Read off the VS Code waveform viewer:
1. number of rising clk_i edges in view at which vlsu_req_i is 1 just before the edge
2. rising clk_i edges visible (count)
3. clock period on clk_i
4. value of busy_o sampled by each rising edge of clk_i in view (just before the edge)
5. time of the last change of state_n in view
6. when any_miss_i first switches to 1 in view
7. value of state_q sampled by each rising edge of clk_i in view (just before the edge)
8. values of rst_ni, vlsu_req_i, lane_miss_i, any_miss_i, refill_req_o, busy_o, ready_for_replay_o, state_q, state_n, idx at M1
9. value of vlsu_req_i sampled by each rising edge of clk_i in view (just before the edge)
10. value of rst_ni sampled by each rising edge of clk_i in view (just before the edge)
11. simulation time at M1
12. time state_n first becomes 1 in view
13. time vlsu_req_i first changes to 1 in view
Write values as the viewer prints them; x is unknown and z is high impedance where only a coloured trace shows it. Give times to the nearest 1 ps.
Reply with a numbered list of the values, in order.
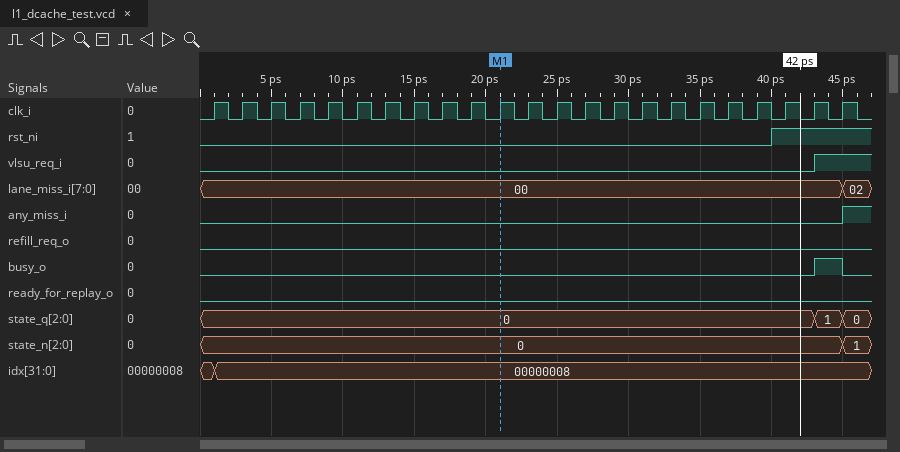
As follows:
1. 1
2. 23
3. 2 ps
4. 0 0 0 0 0 0 0 0 0 0 0 0 0 0 0 0 0 0 0 0 0 0 1
5. 45 ps
6. 45 ps
7. 0, 0, 0, 0, 0, 0, 0, 0, 0, 0, 0, 0, 0, 0, 0, 0, 0, 0, 0, 0, 0, 0, 1
8. rst_ni=0, vlsu_req_i=0, lane_miss_i=00, any_miss_i=0, refill_req_o=0, busy_o=0, ready_for_replay_o=0, state_q=0, state_n=0, idx=00000008
9. 0 0 0 0 0 0 0 0 0 0 0 0 0 0 0 0 0 0 0 0 0 0 1
10. 0 0 0 0 0 0 0 0 0 0 0 0 0 0 0 0 0 0 0 0 1 1 1
11. 21 ps
12. 45 ps
13. 43 ps
